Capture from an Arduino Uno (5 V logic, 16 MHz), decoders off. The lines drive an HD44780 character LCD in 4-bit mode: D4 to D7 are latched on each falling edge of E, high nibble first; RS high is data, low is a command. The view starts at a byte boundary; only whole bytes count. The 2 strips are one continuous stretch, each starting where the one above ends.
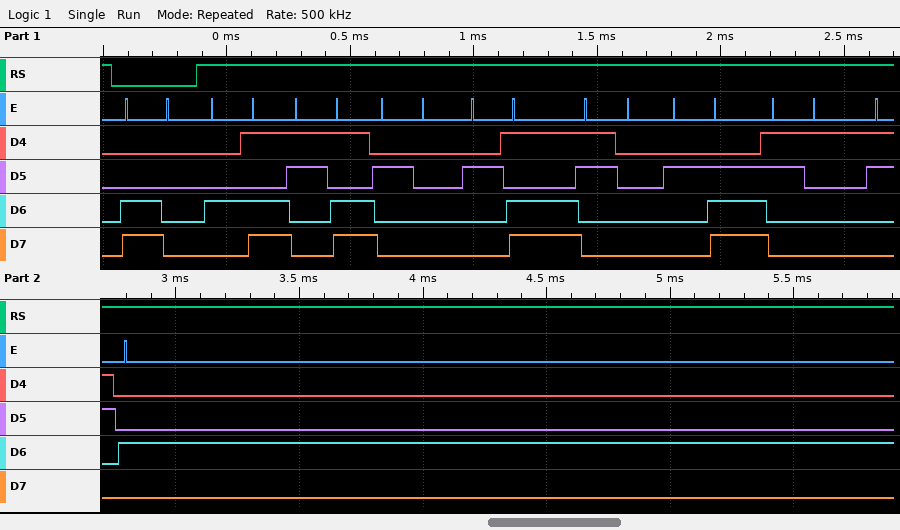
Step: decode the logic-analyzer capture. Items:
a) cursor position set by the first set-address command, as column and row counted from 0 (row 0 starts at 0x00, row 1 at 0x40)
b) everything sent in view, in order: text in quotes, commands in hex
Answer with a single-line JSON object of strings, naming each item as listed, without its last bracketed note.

{"cursor position set by the first set-address command, as column and row counted from 0": "column 0, row 1", "everything sent in view, in order: text in quotes, commands in hex": "0xC0 \"M= -0.14\""}
